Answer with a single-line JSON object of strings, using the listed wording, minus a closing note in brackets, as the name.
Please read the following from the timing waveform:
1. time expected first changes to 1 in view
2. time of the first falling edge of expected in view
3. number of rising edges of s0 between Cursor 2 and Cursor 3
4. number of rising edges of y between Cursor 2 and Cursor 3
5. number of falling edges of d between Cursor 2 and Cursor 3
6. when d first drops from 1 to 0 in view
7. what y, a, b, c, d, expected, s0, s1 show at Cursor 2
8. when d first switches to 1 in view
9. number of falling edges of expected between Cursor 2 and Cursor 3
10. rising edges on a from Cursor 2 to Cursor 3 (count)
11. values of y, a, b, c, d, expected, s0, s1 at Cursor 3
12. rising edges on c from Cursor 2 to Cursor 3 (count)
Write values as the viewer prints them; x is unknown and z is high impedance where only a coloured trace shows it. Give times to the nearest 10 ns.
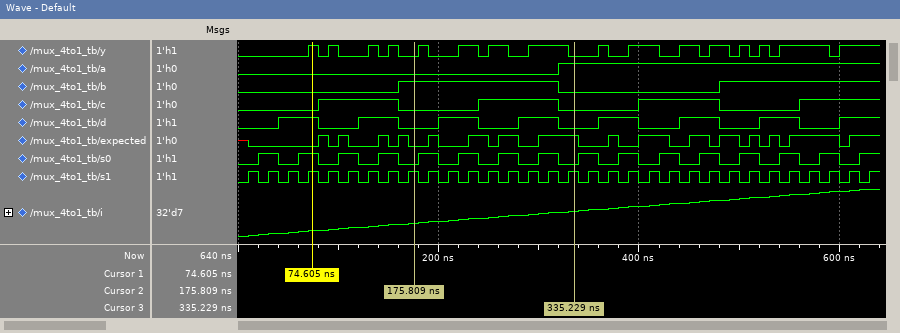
{"time expected first changes to 1 in view": "80 ns", "time of the first falling edge of expected in view": "90 ns", "number of rising edges of s0 between Cursor 2 and Cursor 3": "4", "number of rising edges of y between Cursor 2 and Cursor 3": "4", "number of falling edges of d between Cursor 2 and Cursor 3": "2", "when d first drops from 1 to 0 in view": "80 ns", "what y, a, b, c, d, expected, s0, s1 show at Cursor 2": "y=0, a=0, b=1, c=0, d=0, expected=0, s0=0, s1=1", "when d first switches to 1 in view": "40 ns", "number of falling edges of expected between Cursor 2 and Cursor 3": "3", "rising edges on a from Cursor 2 to Cursor 3": "1", "values of y, a, b, c, d, expected, s0, s1 at Cursor 3": "y=0, a=1, b=0, c=0, d=0, expected=1, s0=0, s1=1", "rising edges on c from Cursor 2 to Cursor 3": "1"}
